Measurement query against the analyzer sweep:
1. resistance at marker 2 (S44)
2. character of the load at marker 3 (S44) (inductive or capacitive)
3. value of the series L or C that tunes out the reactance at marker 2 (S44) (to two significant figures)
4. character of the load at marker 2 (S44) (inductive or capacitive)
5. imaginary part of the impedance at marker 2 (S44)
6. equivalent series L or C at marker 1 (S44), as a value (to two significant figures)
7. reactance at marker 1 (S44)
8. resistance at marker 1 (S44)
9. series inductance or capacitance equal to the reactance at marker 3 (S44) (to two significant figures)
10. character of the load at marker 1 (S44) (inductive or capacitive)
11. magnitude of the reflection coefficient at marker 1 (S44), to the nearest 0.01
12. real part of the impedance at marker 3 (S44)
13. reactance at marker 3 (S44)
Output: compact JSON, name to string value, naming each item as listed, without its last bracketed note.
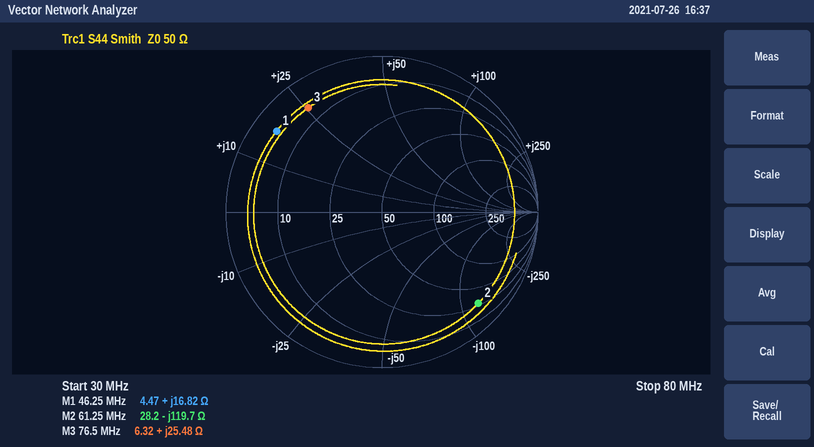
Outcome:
{"resistance at marker 2": "28.2 Ω", "character of the load at marker 3 (S44)": "inductive", "value of the series L or C that tunes out the reactance at marker 2 (S44)": "310 nH", "character of the load at marker 2 (S44)": "capacitive", "imaginary part of the impedance at marker 2": "-119.7 Ω", "equivalent series L or C at marker 1 (S44), as a value": "58 nH", "reactance at marker 1": "+16.82 Ω", "resistance at marker 1": "4.47 Ω", "series inductance or capacitance equal to the reactance at marker 3 (S44)": "53 nH", "character of the load at marker 1 (S44)": "inductive", "magnitude of the reflection coefficient at marker 1 (S44), to the nearest 0.01": "0.85", "real part of the impedance at marker 3": "6.32 Ω", "reactance at marker 3": "+25.48 Ω"}
